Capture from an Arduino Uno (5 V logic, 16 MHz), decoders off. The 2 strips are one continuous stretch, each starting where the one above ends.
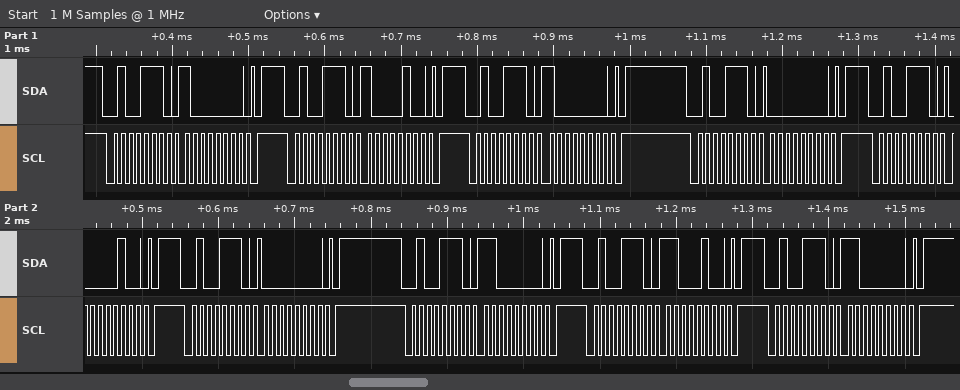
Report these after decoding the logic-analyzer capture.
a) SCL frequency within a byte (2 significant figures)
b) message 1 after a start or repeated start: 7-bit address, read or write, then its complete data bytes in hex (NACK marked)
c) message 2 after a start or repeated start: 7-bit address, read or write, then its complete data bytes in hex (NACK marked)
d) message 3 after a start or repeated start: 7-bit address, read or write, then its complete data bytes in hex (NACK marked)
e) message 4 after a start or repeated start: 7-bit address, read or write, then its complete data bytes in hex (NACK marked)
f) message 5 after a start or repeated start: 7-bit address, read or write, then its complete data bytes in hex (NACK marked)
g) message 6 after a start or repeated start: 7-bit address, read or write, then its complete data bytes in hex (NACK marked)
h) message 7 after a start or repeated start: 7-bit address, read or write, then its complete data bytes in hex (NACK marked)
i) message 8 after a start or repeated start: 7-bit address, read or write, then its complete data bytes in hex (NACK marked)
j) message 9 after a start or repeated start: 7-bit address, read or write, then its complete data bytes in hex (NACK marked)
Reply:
100 kHz
0x27 write: 80
0x27 write: 84
0x27 write: 80
0x27 write: 00
0x27 write: 04
0x27 write: 00
0x27 write: C0
0x27 write: C4
0x27 write: C0
